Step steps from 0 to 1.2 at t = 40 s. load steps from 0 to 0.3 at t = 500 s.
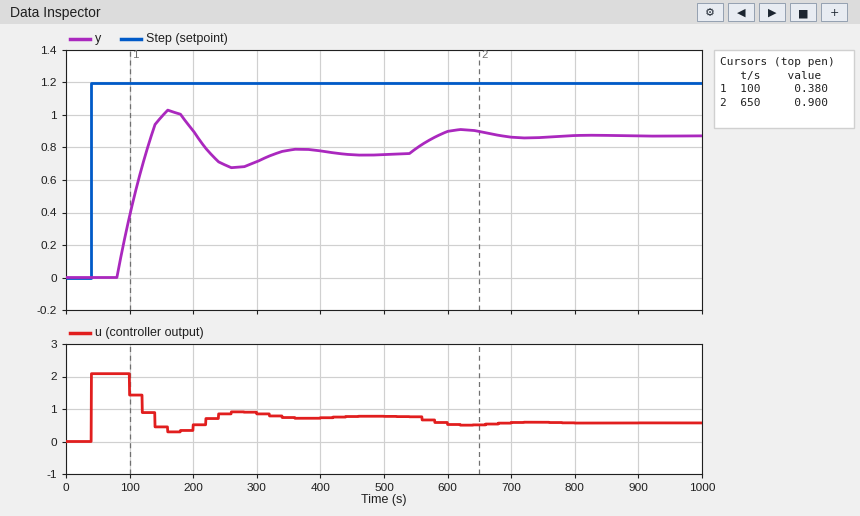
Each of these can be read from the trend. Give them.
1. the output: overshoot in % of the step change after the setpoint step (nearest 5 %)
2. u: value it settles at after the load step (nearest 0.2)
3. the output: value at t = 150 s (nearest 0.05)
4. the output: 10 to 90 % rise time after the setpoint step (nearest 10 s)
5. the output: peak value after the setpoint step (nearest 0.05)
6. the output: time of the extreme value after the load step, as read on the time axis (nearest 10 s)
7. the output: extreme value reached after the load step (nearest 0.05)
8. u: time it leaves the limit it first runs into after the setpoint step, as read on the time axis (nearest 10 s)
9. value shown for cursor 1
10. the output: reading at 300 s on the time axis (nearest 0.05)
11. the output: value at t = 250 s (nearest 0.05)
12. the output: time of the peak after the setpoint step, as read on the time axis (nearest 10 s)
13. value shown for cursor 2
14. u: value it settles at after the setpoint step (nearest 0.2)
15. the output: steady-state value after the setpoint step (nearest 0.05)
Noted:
35 %
0.6
1.00
40 s
1.05
620 s
0.90
100 s
0.380
0.70
0.70
160 s
0.900
0.8
0.75
